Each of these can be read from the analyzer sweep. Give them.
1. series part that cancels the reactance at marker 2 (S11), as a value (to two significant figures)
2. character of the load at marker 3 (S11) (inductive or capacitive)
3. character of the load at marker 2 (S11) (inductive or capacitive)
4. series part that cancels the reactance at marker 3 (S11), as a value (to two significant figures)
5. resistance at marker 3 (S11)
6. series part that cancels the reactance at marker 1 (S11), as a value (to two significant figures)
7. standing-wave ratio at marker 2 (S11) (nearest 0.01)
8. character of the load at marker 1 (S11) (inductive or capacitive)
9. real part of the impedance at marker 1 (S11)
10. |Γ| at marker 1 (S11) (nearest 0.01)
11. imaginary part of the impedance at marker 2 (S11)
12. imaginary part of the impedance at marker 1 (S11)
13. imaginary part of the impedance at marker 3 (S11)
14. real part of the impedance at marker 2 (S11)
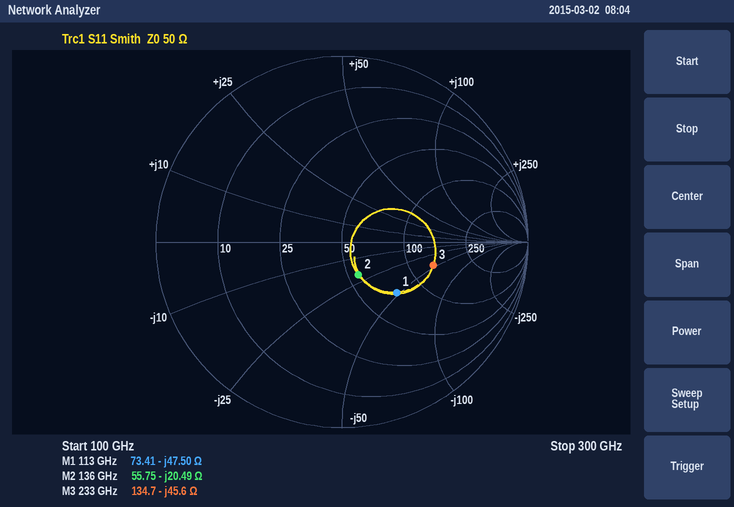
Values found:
24 pH
capacitive
capacitive
31 pH
134.7 Ω
67 pH
1.49
capacitive
73.41 Ω
0.40
-20.49 Ω
-47.50 Ω
-45.6 Ω
55.75 Ω
